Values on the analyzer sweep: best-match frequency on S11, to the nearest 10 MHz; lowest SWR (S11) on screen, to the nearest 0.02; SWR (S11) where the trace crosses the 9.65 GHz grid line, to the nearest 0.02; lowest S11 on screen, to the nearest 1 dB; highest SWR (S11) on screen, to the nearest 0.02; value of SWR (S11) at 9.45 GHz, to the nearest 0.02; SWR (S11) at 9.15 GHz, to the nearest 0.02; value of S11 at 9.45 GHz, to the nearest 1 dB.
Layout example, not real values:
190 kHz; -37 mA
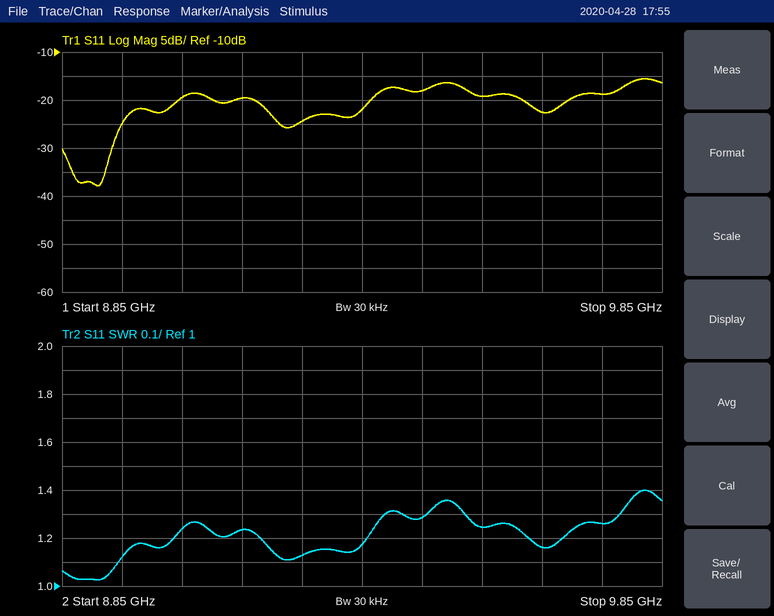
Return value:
8.91 GHz; 1.02; 1.16; -38 dB; 1.40; 1.28; 1.24; -18 dB
